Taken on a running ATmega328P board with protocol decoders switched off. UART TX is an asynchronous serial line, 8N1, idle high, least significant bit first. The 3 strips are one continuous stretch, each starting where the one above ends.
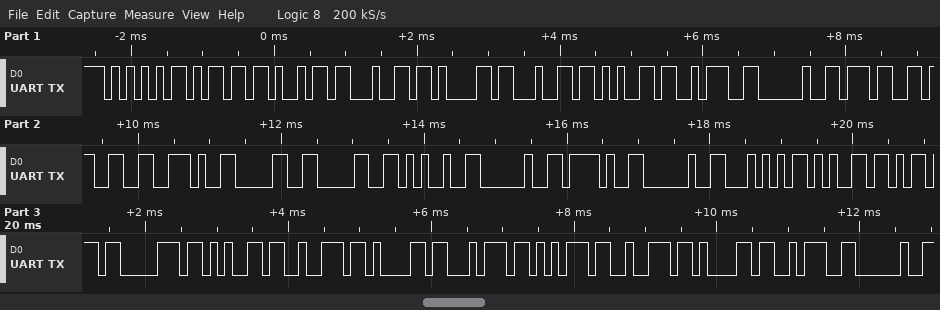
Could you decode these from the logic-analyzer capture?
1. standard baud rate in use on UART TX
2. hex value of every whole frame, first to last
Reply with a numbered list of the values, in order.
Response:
1. 9600 baud
2. 55 6D 69 64 61 64 65 3A 20 37 33 2E 30 30 25 20 2F 20 54 65 6D 70 65 72 61 74 75 72 61 3A 20
